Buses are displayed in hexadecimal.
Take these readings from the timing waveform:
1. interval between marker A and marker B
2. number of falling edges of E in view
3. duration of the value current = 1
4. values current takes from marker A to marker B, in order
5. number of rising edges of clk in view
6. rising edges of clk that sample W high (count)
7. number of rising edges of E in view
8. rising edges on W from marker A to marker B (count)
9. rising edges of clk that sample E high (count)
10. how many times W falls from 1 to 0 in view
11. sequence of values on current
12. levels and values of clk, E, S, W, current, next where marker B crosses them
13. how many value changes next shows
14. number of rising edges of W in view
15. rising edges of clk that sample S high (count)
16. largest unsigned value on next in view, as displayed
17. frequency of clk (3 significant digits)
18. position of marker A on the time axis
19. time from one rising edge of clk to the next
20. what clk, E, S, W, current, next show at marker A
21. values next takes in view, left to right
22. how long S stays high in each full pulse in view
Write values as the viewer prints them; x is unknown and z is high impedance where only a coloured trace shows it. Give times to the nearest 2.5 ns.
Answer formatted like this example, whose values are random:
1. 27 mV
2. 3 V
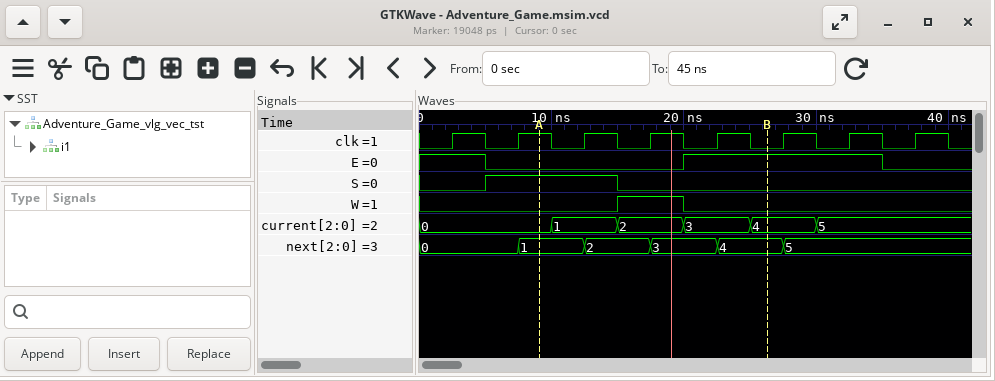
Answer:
1. 17.5 ns
2. 2
3. 5 ns
4. 0, 1, 2, 3, 4
5. 8
6. 1
7. 1
8. 1
9. 4
10. 1
11. 0, 1, 2, 3, 4, 5
12. clk=0, E=1, S=0, W=0, current=4, next=4
13. 5
14. 1
15. 2
16. 5
17. 200 MHz
18. 10 ns
19. 5 ns
20. clk=1, E=0, S=1, W=0, current=0, next=1
21. 0, 1, 2, 3, 4, 5
22. 10 ns
